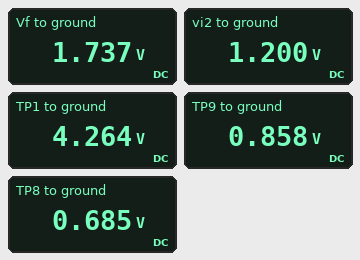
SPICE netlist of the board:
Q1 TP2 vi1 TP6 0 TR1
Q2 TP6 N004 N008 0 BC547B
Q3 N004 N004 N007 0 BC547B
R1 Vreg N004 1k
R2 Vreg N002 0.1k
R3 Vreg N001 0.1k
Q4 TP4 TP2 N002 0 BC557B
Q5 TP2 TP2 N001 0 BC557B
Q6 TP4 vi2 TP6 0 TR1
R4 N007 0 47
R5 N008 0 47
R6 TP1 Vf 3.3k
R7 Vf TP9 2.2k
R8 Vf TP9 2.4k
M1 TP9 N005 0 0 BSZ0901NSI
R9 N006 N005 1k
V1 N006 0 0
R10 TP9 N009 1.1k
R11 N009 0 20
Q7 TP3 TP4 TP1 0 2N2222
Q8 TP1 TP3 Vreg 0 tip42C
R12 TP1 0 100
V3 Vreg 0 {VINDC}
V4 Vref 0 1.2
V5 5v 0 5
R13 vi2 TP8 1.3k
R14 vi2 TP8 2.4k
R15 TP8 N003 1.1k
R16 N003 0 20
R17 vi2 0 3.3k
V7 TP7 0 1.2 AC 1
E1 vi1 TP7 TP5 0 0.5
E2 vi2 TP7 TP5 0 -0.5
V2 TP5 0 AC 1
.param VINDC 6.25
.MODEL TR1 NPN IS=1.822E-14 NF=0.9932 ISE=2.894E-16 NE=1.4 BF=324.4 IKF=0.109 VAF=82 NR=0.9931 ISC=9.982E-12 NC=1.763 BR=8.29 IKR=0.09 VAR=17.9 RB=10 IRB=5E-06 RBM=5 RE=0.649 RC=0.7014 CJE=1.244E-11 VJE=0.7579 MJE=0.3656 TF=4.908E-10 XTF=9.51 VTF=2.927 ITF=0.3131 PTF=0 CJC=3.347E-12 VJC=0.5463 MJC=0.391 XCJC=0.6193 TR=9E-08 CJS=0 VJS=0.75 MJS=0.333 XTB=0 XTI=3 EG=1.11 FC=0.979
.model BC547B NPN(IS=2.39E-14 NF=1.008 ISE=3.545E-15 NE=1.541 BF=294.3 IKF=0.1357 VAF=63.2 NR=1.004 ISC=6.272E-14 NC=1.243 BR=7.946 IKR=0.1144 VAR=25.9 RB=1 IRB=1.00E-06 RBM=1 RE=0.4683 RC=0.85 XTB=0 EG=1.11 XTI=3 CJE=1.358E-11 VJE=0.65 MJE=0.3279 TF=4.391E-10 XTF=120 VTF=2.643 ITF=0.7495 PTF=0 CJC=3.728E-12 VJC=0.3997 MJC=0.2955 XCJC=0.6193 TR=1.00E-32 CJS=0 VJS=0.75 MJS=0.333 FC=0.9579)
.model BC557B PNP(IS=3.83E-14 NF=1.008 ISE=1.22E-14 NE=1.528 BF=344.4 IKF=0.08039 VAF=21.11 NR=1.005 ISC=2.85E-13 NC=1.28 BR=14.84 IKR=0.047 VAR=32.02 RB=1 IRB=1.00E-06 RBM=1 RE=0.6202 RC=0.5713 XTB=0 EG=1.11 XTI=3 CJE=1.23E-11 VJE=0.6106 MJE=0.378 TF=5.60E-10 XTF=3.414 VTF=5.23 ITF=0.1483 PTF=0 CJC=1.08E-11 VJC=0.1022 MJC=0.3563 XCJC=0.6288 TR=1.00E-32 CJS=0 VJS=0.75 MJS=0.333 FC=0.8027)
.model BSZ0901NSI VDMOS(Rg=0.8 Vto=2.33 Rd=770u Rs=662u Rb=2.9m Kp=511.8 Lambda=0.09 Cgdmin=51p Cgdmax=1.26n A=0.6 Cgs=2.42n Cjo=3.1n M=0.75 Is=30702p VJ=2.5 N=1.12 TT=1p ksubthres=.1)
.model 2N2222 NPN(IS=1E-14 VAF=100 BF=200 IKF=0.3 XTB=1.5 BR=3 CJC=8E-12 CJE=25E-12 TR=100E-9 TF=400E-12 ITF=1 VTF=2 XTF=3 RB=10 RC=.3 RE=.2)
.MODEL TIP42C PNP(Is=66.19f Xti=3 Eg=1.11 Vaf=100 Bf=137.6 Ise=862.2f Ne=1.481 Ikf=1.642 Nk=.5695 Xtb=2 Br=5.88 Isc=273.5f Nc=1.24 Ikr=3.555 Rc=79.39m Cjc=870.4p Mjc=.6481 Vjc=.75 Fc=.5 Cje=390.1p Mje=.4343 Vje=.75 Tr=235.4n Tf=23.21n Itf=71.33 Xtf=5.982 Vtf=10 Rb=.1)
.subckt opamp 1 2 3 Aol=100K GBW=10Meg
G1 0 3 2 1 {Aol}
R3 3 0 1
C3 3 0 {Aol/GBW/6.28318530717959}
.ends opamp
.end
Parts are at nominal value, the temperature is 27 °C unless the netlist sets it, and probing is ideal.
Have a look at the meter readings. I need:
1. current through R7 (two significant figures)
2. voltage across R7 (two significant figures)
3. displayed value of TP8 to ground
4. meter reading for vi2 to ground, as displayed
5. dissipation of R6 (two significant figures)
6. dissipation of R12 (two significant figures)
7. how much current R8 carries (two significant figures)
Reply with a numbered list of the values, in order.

1. 400 µA
2. 880 mV
3. 0.685 V
4. 1.200 V
5. 1.9 mW
6. 180 mW
7. 370 µA
